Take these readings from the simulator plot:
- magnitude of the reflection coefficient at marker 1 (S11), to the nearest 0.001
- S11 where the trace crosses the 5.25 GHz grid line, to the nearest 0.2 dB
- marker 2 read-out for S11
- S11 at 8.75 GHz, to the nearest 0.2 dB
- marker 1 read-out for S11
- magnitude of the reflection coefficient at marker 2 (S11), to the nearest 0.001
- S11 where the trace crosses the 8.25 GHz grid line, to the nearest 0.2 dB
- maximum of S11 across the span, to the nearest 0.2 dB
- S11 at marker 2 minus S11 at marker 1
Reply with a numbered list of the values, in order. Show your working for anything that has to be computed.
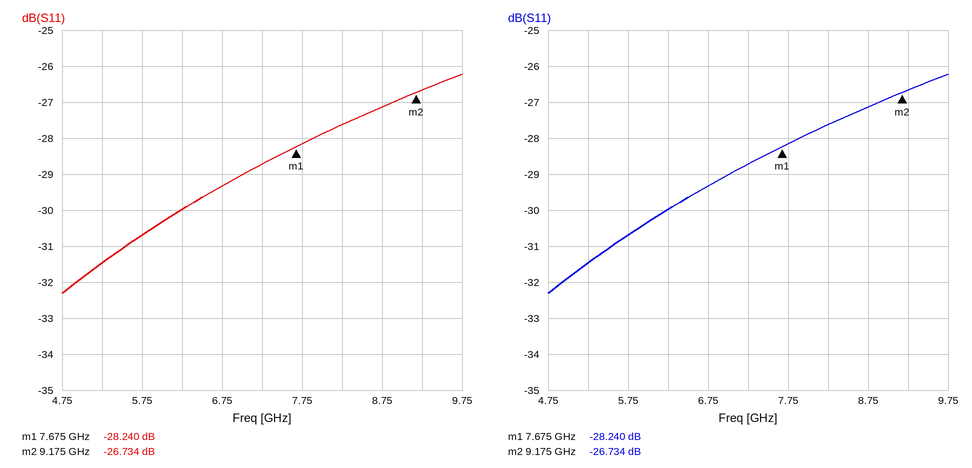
1. 10^(-28.24/20) ≈ 0.039
2. -31.4 dB
3. -26.734 dB
4. -27.2 dB
5. -28.240 dB
6. 10^(-26.734/20) ≈ 0.046
7. -27.6 dB
8. -26.2 dB
9. -26.734 − (-28.24) = 1.506 dB
